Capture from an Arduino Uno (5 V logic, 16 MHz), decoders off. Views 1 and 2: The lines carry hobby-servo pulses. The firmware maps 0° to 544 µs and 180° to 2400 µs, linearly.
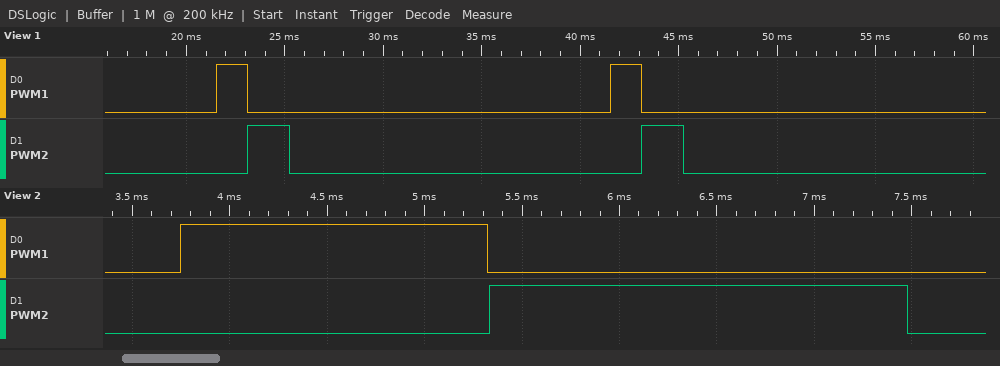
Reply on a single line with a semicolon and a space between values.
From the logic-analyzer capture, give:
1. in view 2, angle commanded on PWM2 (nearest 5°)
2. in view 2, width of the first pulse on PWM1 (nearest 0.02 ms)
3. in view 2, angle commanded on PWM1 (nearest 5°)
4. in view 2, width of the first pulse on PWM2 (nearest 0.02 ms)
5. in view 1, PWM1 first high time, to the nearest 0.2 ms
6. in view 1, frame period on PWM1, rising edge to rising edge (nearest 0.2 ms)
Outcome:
155°; 1.58 ms; 100°; 2.14 ms; 1.6 ms; 20.0 ms
